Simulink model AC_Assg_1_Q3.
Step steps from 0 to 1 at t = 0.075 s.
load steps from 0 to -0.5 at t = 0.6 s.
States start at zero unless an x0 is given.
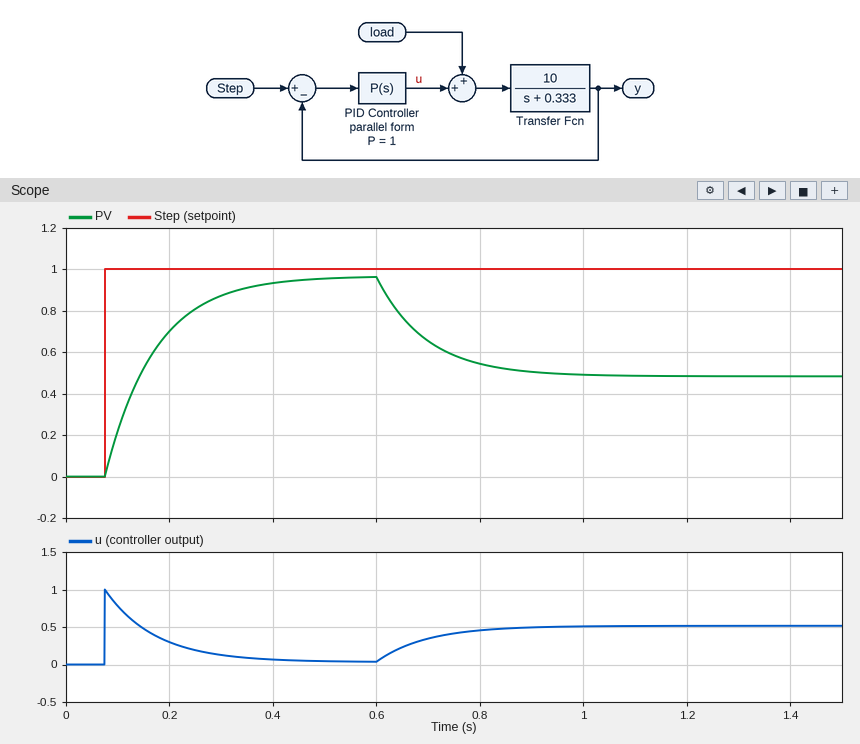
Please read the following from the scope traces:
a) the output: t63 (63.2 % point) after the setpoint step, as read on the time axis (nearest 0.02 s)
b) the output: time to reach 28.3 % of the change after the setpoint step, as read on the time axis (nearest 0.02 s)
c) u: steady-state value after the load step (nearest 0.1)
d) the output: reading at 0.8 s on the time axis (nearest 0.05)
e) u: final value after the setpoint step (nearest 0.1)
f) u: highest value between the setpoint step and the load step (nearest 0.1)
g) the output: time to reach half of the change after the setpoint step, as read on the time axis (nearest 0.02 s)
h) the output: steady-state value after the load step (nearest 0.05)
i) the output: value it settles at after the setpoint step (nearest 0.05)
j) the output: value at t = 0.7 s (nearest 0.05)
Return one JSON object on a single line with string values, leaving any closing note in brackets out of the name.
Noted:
{"the output: t63 (63.2 % point) after the setpoint step, as read on the time axis": "0.18 s", "the output: time to reach 28.3 % of the change after the setpoint step, as read on the time axis": "0.10 s", "u: steady-state value after the load step": "0.5", "the output: reading at 0.8 s on the time axis": "0.55", "u: final value after the setpoint step": "0.0", "u: highest value between the setpoint step and the load step": "1.0", "the output: time to reach half of the change after the setpoint step, as read on the time axis": "0.14 s", "the output: steady-state value after the load step": "0.50", "the output: value it settles at after the setpoint step": "0.95", "the output: value at t = 0.7 s": "0.65"}
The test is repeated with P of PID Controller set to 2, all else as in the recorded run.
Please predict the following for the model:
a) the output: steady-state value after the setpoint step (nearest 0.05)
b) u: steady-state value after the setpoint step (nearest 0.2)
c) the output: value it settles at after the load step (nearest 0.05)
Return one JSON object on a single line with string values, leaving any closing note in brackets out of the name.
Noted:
{"the output: steady-state value after the setpoint step": "1.00", "u: steady-state value after the setpoint step": "0.0", "the output: value it settles at after the load step": "0.75"}
